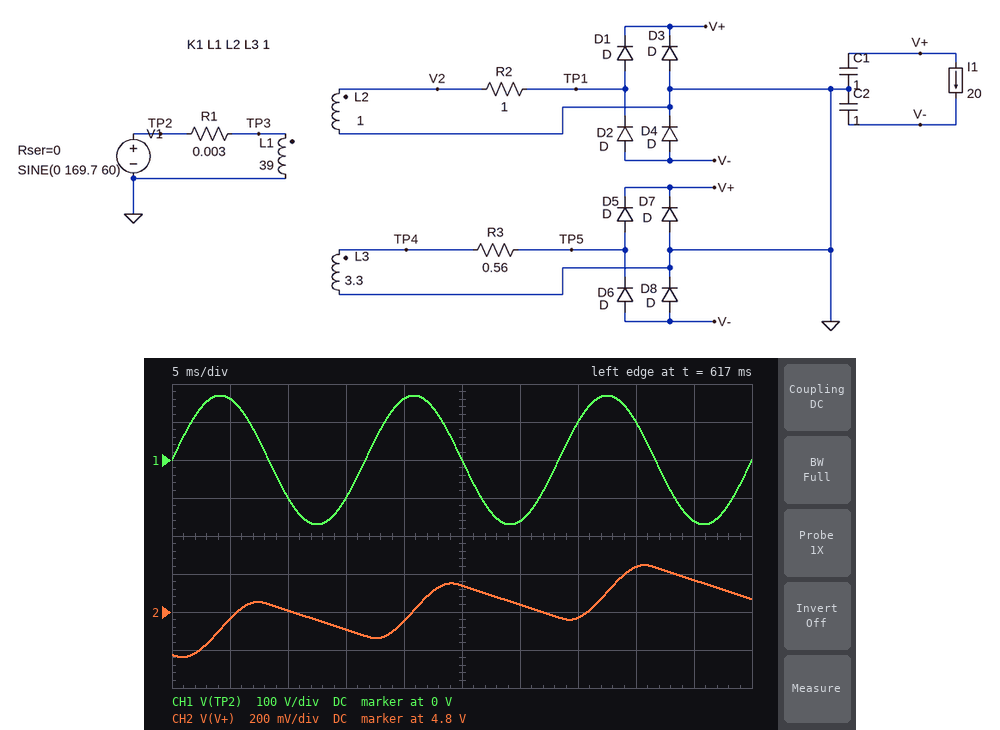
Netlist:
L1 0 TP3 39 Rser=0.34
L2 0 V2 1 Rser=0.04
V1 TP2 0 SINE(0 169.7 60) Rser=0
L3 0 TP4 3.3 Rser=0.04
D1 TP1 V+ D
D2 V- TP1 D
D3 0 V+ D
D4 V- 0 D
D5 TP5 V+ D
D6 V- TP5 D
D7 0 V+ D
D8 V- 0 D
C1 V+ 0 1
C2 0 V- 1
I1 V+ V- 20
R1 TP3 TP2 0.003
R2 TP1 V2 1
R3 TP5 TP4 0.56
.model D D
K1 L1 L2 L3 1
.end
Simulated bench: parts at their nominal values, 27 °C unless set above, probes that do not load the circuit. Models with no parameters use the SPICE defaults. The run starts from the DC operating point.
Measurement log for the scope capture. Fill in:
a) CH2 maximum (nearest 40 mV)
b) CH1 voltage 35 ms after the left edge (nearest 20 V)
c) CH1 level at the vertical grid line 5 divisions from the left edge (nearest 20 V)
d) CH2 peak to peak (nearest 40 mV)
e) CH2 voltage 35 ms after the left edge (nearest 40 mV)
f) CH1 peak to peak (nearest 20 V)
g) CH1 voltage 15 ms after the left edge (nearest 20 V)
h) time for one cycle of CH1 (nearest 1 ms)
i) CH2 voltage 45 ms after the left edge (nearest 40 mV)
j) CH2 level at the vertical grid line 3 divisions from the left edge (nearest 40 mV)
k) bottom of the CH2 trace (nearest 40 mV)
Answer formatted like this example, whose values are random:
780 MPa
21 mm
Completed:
5.04 V
100 V
0 V
480 mV
4.76 V
340 V
-100 V
17 ms
4.96 V
4.72 V
4.56 V
